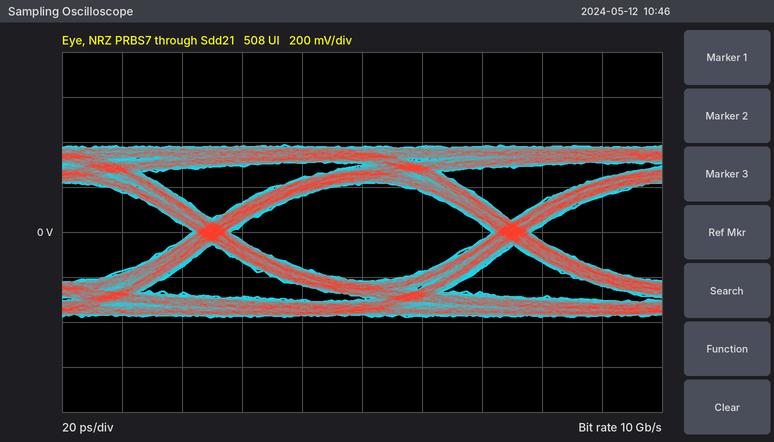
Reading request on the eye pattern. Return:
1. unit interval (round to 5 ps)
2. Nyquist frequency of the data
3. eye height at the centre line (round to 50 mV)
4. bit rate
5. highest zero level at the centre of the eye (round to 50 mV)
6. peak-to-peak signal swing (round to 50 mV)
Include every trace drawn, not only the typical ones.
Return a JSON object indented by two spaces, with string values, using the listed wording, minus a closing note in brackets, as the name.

{
  "unit interval": "100 ps",
  "Nyquist frequency of the data": "5 GHz",
  "eye height at the centre line": "450 mV",
  "bit rate": "10 Gb/s",
  "highest zero level at the centre of the eye": "-200 mV",
  "peak-to-peak signal swing": "750 mV"
}
